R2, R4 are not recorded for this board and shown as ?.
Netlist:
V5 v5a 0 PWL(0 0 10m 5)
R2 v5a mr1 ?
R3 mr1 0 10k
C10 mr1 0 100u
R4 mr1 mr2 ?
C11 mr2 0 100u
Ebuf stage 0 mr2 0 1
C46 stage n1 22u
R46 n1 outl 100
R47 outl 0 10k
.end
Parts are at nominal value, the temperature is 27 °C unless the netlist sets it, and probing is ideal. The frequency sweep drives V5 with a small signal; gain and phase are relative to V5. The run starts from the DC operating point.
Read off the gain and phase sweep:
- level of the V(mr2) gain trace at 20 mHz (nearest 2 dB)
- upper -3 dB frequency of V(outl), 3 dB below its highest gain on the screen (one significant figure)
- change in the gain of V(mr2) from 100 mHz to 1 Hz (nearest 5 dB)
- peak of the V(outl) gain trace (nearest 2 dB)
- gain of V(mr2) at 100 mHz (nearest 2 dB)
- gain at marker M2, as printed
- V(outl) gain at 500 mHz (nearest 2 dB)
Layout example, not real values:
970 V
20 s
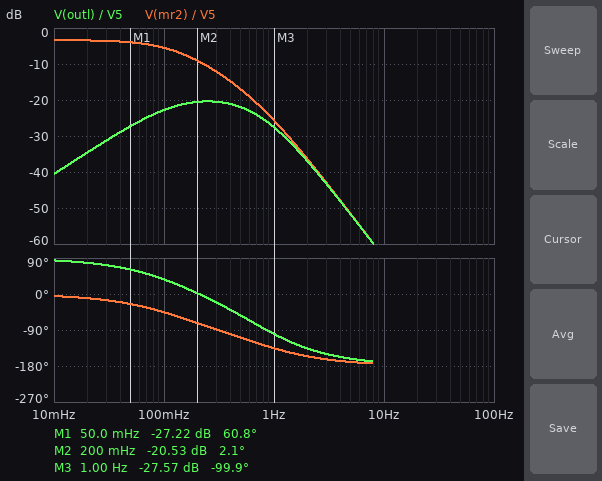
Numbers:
-4 dB
600 mHz
-20 dB
-20 dB
-6 dB
-20.53 dB
-22 dB
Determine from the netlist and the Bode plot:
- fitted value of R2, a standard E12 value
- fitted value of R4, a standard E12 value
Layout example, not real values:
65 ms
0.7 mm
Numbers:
4.7 kΩ
8.2 kΩ
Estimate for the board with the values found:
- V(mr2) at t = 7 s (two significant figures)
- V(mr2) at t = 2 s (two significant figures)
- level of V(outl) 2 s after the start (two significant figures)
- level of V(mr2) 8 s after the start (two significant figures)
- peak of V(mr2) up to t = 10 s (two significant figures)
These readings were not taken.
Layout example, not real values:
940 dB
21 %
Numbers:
3.4 V
2.6 V
180 mV
3.4 V
3.4 V
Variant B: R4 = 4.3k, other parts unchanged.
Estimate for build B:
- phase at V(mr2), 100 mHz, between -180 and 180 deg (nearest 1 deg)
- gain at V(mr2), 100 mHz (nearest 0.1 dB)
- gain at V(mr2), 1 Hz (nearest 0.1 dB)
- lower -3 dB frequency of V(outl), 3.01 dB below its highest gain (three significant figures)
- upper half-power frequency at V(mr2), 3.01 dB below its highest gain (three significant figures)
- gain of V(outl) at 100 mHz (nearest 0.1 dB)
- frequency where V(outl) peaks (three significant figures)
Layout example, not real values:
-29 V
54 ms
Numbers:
-35 deg
-4.6 dB
-21.5 dB
115 mHz
169 mHz
-21.9 dB
311 mHz
